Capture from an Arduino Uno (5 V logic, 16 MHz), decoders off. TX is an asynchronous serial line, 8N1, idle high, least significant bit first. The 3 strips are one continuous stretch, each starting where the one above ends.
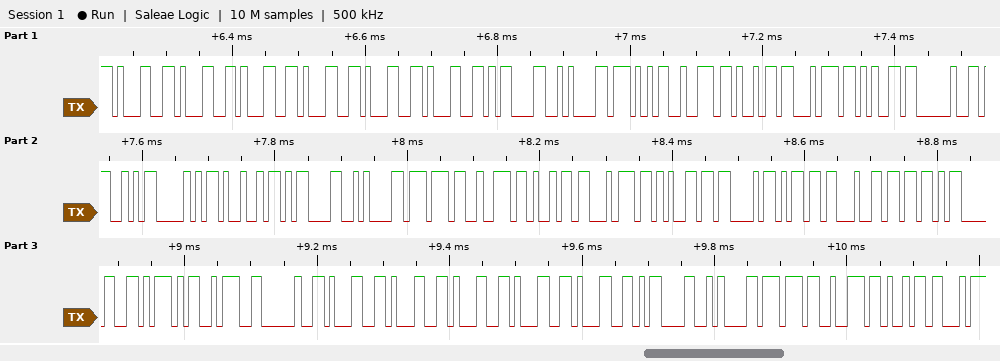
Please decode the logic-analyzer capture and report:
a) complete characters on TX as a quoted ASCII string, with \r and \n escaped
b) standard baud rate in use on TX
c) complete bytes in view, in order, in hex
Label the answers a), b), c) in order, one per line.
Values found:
a) "111111\r\nWrite SPI\r\nwriteCmd[0]: 11111\r\nwri"
b) 115200 baud
c) 31 31 31 31 31 31 0D 0A 57 72 69 74 65 20 53 50 49 0D 0A 77 72 69 74 65 43 6D 64 5B 30 5D 3A 20 31 31 31 31 31 0D 0A 77 72 69
